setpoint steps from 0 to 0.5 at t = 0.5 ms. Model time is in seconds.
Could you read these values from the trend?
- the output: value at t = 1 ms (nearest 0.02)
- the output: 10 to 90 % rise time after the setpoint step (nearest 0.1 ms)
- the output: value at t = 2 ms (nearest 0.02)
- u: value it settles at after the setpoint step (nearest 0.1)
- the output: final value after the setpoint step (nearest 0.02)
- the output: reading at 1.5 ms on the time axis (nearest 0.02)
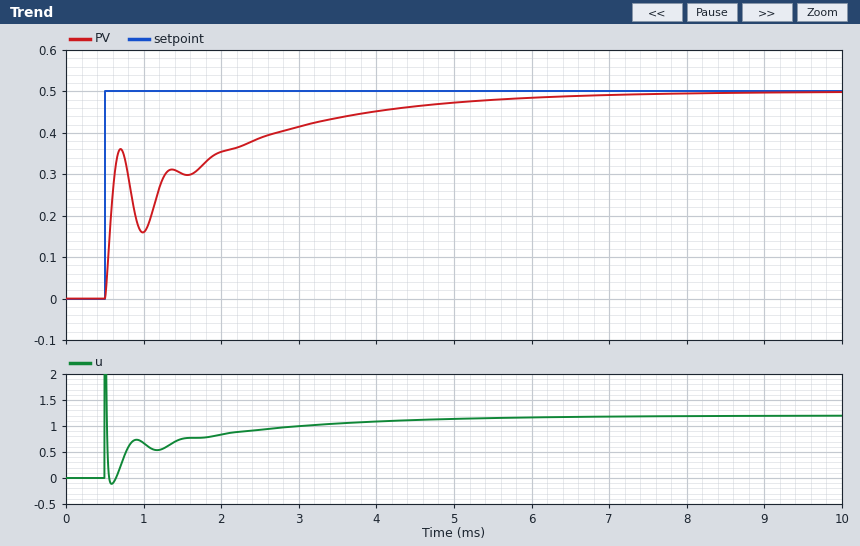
0.16
3.4 ms
0.36
1.2
0.50
0.30
